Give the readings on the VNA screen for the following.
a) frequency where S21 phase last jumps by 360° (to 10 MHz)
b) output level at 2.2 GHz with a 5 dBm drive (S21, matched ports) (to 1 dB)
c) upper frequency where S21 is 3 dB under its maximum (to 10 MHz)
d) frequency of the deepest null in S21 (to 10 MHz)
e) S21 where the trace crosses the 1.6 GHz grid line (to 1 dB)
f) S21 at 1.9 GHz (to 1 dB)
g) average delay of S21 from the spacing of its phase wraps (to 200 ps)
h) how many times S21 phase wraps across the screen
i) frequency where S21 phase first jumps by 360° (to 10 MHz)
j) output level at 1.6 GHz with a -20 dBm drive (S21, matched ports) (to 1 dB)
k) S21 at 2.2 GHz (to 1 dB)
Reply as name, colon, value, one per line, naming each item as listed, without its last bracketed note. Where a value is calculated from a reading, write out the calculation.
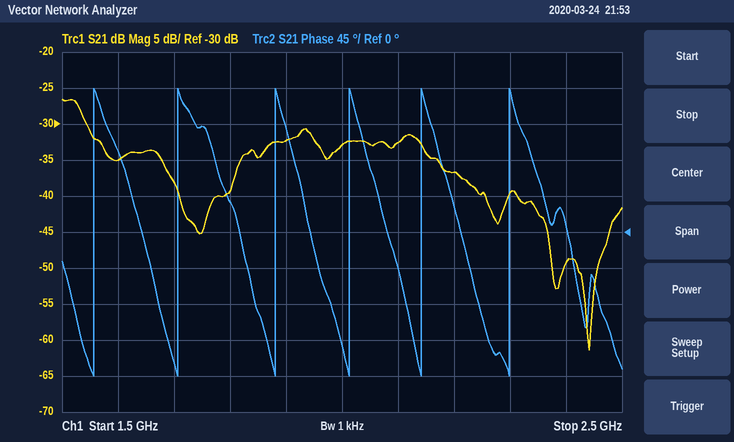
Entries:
frequency where S21 phase last jumps by 360°: 2.30 GHz
output level at 2.2 GHz with a 5 dBm drive (S21, matched ports): 5 dBm + (-37 dB) = -32 dBm
upper frequency where S21 is 3 dB under its maximum: 1.54 GHz
frequency of the deepest null in S21: 2.44 GHz
S21 where the trace crosses the 1.6 GHz grid line: -35 dB
S21 at 1.9 GHz: -32 dB
average delay of S21 from the spacing of its phase wraps: 5 cycles / (2.30 GHz − 1.56 GHz) ≈ 6.8 ns
how many times S21 phase wraps across the screen: 6
frequency where S21 phase first jumps by 360°: 1.56 GHz
output level at 1.6 GHz with a -20 dBm drive (S21, matched ports): -20 dBm + (-35 dB) = -55 dBm
S21 at 2.2 GHz: -37 dB
